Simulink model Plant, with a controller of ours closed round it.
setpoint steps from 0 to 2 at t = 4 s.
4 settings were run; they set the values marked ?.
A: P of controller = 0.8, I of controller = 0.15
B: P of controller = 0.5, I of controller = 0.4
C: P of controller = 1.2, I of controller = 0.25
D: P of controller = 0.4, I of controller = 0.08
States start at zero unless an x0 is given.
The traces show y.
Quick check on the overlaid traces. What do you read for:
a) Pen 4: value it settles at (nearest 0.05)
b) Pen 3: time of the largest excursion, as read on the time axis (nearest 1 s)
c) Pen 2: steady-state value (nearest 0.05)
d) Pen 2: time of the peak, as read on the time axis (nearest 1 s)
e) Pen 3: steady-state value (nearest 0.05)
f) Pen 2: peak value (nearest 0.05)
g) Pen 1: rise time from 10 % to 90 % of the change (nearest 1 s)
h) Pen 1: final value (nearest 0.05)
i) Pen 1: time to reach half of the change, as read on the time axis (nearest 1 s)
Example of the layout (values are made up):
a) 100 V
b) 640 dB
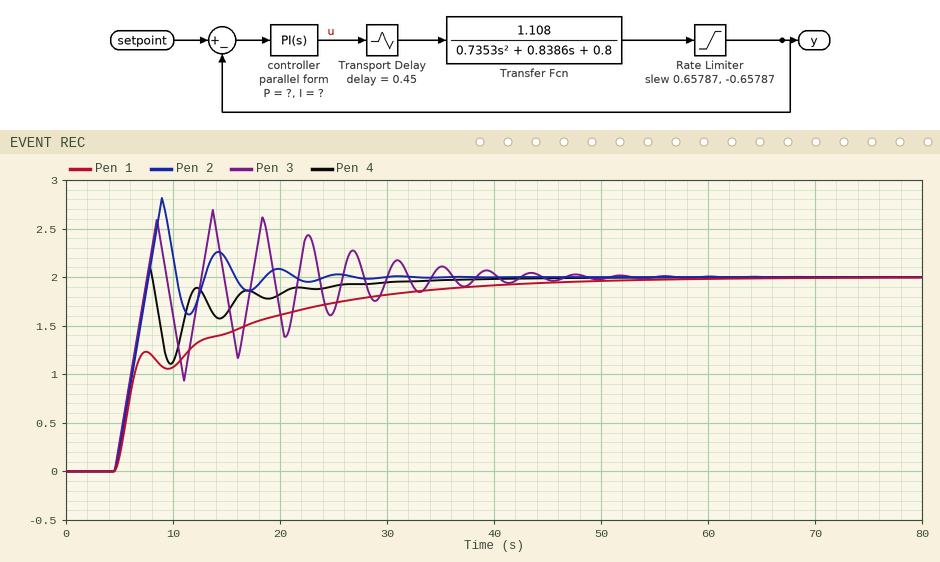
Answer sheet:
a) 2.00
b) 14 s
c) 2.00
d) 9 s
e) 2.00
f) 2.80
g) 24 s
h) 2.00
i) 6 s
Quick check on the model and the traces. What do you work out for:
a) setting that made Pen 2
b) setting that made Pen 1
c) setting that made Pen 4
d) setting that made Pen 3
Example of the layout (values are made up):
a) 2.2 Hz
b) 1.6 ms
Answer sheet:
a) B
b) D
c) A
d) C
